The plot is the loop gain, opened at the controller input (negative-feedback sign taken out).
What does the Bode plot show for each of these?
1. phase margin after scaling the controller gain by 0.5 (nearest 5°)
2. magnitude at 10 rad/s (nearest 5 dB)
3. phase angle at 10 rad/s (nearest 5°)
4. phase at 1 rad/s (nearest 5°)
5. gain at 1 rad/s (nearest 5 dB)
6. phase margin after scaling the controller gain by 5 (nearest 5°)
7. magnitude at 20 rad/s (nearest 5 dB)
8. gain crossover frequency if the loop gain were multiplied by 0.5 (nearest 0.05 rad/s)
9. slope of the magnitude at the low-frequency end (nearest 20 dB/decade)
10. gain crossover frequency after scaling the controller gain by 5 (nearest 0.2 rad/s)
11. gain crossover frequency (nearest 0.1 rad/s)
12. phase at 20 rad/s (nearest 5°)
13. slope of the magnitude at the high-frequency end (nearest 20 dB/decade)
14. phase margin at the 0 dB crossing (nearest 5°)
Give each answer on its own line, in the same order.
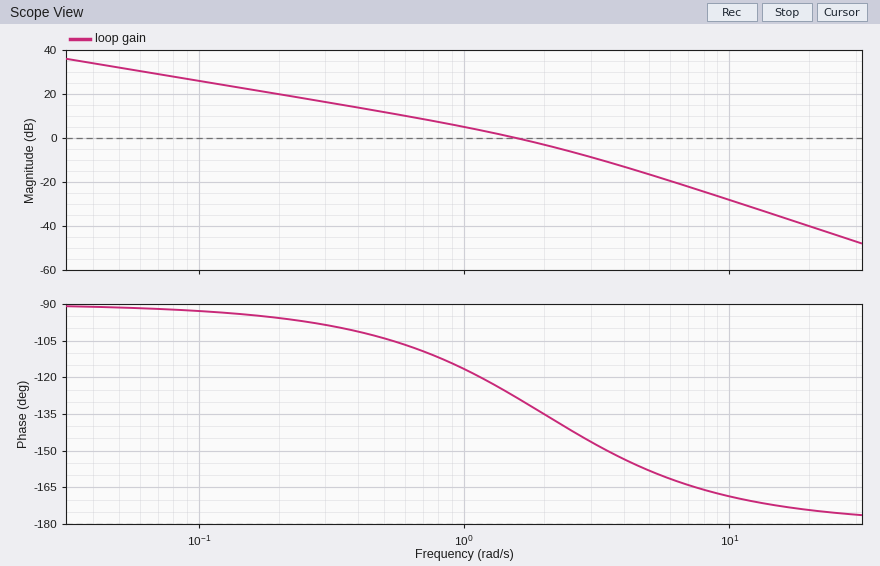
65°
-30 dB
-170°
-115°
5 dB
25°
-40 dB
0.90 rad/s
-20 dB/decade
4.2 rad/s
1.6 rad/s
-175°
-40 dB/decade
50°
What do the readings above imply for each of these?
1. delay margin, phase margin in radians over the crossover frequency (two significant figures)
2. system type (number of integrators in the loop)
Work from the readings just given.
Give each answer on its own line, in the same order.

0.55 s
1
